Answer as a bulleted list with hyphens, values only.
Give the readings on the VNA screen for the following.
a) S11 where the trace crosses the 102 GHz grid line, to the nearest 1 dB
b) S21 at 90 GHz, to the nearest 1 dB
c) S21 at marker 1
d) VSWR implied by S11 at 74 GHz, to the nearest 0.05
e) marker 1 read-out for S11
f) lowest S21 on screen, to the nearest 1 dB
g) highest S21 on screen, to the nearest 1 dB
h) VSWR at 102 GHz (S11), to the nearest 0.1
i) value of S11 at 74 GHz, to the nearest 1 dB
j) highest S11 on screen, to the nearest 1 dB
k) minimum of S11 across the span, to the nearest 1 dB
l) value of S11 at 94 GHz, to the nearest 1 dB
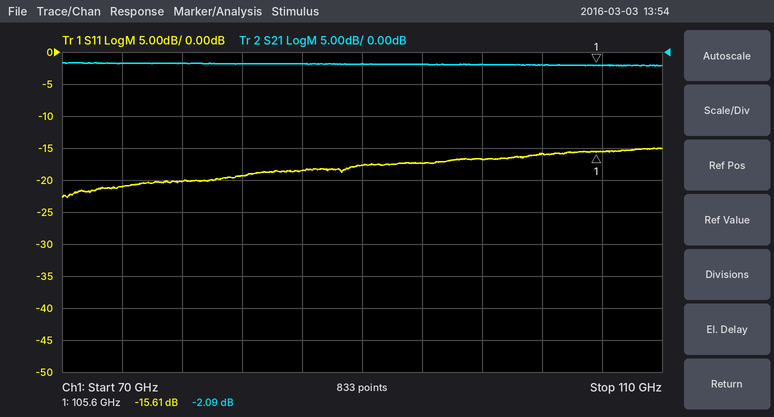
- -16 dB
- -2 dB
- -2.09 dB
- 1.20
- -15.61 dB
- -2 dB
- -2 dB
- 1.4
- -21 dB
- -15 dB
- -23 dB
- -17 dB
